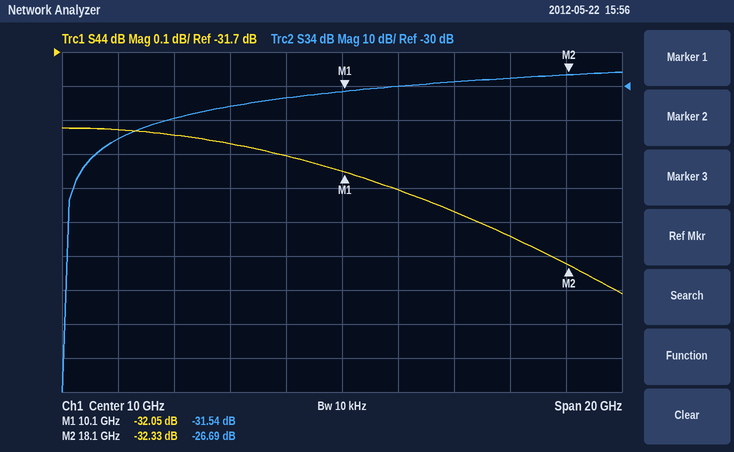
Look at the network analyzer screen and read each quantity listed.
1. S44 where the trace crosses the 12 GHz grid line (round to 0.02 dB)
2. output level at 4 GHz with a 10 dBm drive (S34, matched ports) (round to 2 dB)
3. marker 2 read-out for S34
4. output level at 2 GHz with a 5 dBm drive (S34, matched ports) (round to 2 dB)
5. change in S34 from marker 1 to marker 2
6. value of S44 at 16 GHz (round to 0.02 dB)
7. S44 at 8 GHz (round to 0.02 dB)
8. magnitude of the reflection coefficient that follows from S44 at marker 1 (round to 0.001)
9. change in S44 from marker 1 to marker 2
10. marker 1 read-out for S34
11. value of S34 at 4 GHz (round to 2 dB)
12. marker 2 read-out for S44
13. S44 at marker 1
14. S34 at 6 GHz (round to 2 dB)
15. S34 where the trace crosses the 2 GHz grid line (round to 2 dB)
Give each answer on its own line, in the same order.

-32.10 dB
-30 dBm
-26.69 dB
-40 dBm
4.85 dB
-32.24 dB
-32.00 dB
0.025
-0.28 dB
-31.54 dB
-40 dB
-32.33 dB
-32.05 dB
-36 dB
-46 dB
